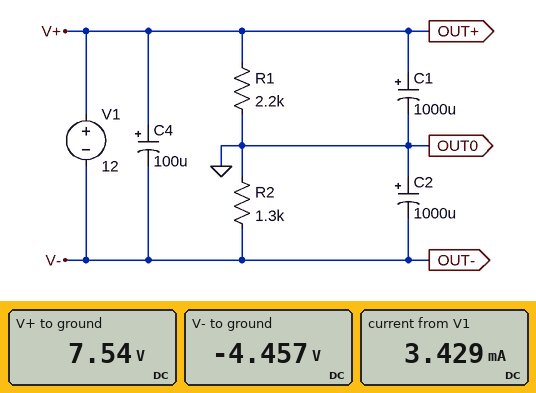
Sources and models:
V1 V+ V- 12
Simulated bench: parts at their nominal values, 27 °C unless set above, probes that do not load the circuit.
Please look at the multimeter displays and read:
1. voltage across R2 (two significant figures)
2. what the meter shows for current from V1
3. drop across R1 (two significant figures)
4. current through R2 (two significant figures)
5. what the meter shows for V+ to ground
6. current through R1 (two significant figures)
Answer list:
4.5 V
3.429 mA
7.5 V
3.4 mA
7.54 V
3.4 mA
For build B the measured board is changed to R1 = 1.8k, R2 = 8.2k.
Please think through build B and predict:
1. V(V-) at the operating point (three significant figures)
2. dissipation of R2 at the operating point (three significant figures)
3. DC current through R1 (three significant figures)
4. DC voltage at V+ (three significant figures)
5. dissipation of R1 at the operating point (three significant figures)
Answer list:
-9.84 V
11.8 mW
1.20 mA
2.16 V
2.59 mW
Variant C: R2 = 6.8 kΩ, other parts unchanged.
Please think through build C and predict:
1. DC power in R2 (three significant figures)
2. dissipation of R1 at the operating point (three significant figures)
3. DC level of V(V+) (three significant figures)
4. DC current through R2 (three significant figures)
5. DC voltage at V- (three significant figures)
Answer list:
12.1 mW
3.91 mW
2.93 V
1.33 mA
-9.07 V
